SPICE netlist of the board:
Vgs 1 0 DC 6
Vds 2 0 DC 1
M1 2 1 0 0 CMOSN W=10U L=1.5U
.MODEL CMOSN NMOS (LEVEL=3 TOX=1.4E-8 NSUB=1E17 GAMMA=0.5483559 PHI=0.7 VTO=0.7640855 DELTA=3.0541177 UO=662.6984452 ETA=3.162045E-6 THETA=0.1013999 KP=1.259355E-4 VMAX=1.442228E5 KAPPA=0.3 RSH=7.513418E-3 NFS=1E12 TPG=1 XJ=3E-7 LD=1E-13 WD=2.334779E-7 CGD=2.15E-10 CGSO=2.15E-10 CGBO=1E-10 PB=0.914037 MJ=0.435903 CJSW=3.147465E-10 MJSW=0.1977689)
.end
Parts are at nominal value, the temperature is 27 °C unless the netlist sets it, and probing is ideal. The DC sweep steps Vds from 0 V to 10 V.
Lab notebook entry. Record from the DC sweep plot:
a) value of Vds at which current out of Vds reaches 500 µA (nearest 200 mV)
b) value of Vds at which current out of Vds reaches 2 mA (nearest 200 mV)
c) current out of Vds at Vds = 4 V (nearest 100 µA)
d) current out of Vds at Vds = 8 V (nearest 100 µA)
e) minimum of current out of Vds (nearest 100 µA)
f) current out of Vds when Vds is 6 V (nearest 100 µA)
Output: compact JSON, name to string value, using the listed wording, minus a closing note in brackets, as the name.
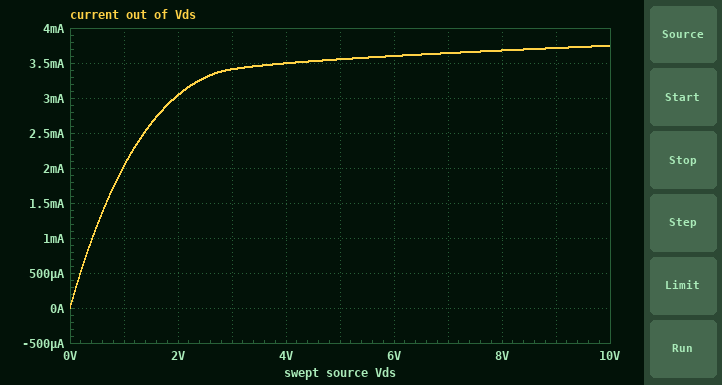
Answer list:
{"value of Vds at which current out of Vds reaches 500 µA": "200 mV", "value of Vds at which current out of Vds reaches 2 mA": "1.0 V", "current out of Vds at Vds = 4 V": "3.5 mA", "current out of Vds at Vds = 8 V": "3.7 mA", "minimum of current out of Vds": "0 A", "current out of Vds when Vds is 6 V": "3.6 mA"}
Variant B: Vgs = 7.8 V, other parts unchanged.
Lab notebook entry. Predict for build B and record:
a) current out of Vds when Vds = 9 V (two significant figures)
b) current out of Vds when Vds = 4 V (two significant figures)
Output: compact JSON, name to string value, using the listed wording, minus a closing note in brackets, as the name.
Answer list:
{"current out of Vds when Vds = 9 V": "5.5 mA", "current out of Vds when Vds = 4 V": "5.1 mA"}
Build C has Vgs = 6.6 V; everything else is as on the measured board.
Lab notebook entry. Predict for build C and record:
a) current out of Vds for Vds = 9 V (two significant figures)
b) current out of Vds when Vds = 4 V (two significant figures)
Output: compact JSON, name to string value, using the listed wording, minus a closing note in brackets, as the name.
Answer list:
{"current out of Vds for Vds = 9 V": "4.3 mA", "current out of Vds when Vds = 4 V": "4.0 mA"}
